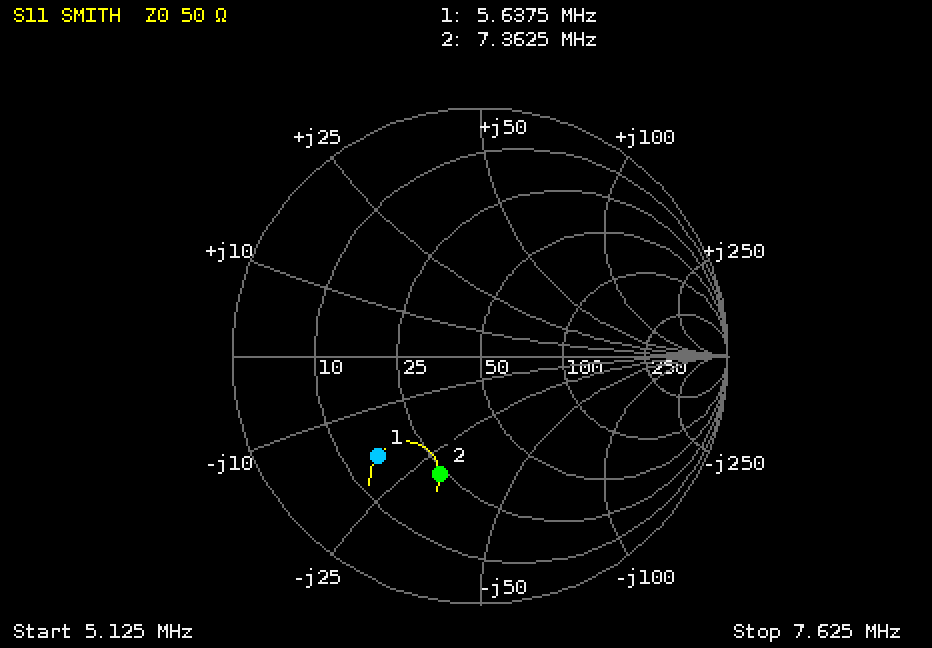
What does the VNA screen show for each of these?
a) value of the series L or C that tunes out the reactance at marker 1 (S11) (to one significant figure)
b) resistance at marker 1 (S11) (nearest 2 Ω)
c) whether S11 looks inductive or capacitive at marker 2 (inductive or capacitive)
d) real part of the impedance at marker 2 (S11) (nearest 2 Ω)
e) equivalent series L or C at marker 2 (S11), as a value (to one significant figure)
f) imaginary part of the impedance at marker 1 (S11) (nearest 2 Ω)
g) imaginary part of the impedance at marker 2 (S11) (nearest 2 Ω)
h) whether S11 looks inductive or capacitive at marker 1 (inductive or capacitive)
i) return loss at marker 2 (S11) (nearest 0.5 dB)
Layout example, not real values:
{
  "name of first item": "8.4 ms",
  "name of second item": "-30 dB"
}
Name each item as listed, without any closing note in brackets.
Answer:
{
  "value of the series L or C that tunes out the reactance at marker 1 (S11)": "500 nH",
  "resistance at marker 1 (S11)": "16 Ω",
  "whether S11 looks inductive or capacitive at marker 2": "capacitive",
  "real part of the impedance at marker 2 (S11)": "24 Ω",
  "equivalent series L or C at marker 2 (S11), as a value": "700 pF",
  "imaginary part of the impedance at marker 1 (S11)": "-18 Ω",
  "imaginary part of the impedance at marker 2 (S11)": "-30 Ω",
  "whether S11 looks inductive or capacitive at marker 1": "capacitive",
  "return loss at marker 2 (S11)": "6.0 dB"
}
